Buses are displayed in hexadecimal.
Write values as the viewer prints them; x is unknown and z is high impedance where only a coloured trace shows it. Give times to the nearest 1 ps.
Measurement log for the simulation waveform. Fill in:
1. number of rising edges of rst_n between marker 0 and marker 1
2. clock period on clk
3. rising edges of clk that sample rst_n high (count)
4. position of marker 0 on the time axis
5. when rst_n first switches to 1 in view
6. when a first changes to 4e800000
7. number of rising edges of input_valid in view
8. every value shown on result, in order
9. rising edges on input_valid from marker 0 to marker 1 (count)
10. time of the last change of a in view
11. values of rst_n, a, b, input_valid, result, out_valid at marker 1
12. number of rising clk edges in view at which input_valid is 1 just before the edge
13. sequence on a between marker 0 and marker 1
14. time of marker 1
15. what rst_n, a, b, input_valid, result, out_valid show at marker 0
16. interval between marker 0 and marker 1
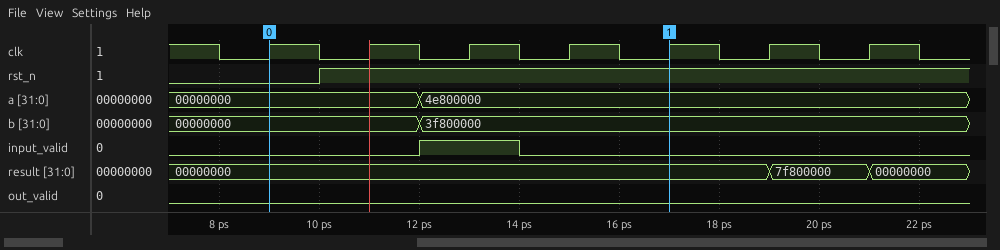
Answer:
1
2 ps
6
9 ps
10 ps
12 ps
1
00000000, 7f800000, 00000000
1
12 ps
rst_n=1, a=4e800000, b=3f800000, input_valid=0, result=00000000, out_valid=0
1
00000000, 4e800000
17 ps
rst_n=0, a=00000000, b=00000000, input_valid=0, result=00000000, out_valid=0
8 ps
